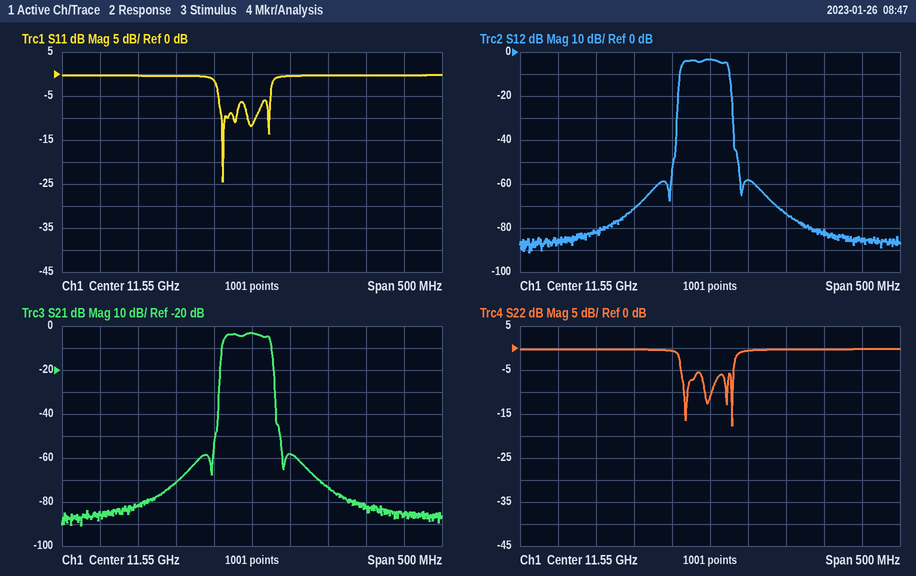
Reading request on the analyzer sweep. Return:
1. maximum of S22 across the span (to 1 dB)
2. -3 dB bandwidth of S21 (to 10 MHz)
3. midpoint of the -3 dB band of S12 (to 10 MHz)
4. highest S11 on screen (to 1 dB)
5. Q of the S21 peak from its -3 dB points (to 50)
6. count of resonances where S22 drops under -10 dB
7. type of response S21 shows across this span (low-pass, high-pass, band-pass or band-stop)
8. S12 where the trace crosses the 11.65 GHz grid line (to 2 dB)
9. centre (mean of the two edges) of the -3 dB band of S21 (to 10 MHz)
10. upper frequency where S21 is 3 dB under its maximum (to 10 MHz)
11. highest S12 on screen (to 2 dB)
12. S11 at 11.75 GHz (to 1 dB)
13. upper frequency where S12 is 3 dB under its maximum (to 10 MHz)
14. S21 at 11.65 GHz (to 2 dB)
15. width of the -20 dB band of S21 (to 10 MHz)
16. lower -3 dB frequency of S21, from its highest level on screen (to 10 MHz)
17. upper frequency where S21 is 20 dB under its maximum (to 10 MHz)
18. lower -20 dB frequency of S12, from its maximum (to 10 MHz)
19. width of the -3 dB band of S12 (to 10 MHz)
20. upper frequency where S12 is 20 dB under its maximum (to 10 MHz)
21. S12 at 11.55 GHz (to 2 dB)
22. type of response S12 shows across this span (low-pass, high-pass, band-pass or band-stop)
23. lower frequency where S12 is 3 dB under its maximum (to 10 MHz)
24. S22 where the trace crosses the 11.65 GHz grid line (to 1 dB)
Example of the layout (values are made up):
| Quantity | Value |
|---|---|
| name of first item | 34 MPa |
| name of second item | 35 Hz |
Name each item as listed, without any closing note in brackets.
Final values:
| Quantity | Value |
|---|---|
| maximum of S22 across the span | 0 dB |
| -3 dB bandwidth of S21 | 60 MHz |
| midpoint of the -3 dB band of S12 | 11.54 GHz |
| highest S11 on screen | 0 dB |
| Q of the S21 peak from its -3 dB points | 200 |
| count of resonances where S22 drops under -10 dB | 4 |
| type of response S21 shows across this span | band-pass |
| S12 where the trace crosses the 11.65 GHz grid line | -74 dB |
| centre (mean of the two edges) of the -3 dB band of S21 | 11.54 GHz |
| upper frequency where S21 is 3 dB under its maximum | 11.57 GHz |
| highest S12 on screen | -4 dB |
| S11 at 11.75 GHz | 0 dB |
| upper frequency where S12 is 3 dB under its maximum | 11.57 GHz |
| S21 at 11.65 GHz | -74 dB |
| width of the -20 dB band of S21 | 70 MHz |
| lower -3 dB frequency of S21, from its highest level on screen | 11.51 GHz |
| upper frequency where S21 is 20 dB under its maximum | 11.58 GHz |
| lower -20 dB frequency of S12, from its maximum | 11.51 GHz |
| width of the -3 dB band of S12 | 60 MHz |
| upper frequency where S12 is 20 dB under its maximum | 11.58 GHz |
| S12 at 11.55 GHz | -4 dB |
| type of response S12 shows across this span | band-pass |
| lower frequency where S12 is 3 dB under its maximum | 11.51 GHz |
| S22 where the trace crosses the 11.65 GHz grid line | 0 dB |
